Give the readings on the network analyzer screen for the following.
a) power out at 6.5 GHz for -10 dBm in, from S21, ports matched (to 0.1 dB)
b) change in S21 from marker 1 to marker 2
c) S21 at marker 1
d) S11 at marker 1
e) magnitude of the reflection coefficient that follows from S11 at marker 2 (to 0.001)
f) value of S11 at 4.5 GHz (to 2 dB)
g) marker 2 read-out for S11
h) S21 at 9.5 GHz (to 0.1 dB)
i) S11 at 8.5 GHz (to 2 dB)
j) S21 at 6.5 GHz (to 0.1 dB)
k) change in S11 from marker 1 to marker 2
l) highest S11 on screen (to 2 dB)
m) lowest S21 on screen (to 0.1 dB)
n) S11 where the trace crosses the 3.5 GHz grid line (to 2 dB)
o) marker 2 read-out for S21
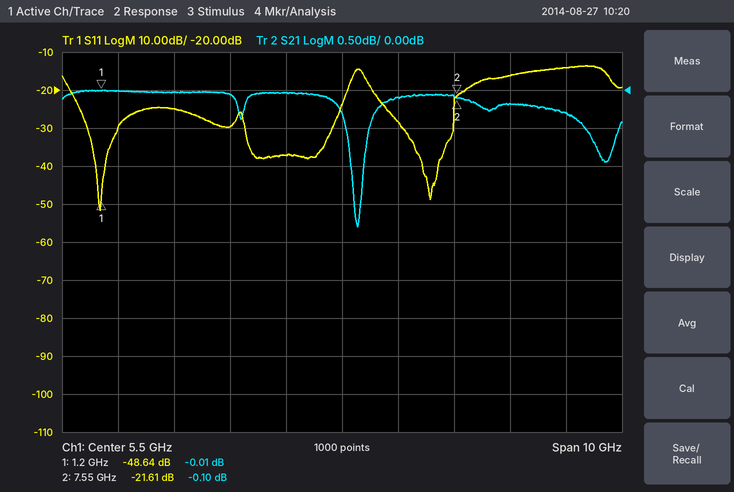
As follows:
-10.1 dBm
-0.09 dB
-0.01 dB
-48.64 dB
0.083
-38 dB
-21.61 dB
-0.3 dB
-16 dB
-0.1 dB
27.03 dB
-14 dB
-1.8 dB
-30 dB
-0.10 dB
